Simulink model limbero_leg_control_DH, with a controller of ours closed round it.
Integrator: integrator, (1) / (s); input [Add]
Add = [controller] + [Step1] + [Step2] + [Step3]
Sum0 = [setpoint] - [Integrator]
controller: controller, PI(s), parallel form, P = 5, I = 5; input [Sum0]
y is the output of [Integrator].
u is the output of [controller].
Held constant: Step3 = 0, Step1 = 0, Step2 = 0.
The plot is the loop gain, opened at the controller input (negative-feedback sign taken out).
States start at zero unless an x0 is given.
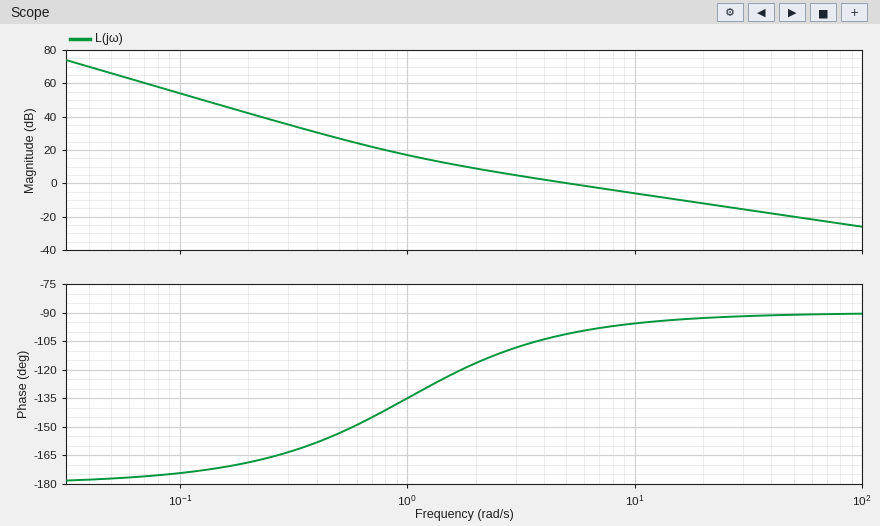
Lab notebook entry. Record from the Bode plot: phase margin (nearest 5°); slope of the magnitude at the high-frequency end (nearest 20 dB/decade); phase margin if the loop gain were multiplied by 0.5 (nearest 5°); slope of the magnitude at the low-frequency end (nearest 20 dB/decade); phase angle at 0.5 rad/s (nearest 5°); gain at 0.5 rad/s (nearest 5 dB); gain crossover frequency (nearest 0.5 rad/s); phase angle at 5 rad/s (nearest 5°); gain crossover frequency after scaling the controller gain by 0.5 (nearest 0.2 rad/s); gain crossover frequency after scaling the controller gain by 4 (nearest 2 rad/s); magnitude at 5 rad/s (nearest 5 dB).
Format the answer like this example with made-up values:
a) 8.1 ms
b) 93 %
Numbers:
a) 80°
b) -20 dB/decade
c) 70°
d) -40 dB/decade
e) -155°
f) 25 dB
g) 5.0 rad/s
h) -100°
i) 2.6 rad/s
j) 20 rad/s
k) 0 dB
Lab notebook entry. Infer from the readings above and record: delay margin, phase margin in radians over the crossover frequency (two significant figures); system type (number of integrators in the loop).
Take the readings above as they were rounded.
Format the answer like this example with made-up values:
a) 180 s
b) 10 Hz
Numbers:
a) 0.28 s
b) 2
